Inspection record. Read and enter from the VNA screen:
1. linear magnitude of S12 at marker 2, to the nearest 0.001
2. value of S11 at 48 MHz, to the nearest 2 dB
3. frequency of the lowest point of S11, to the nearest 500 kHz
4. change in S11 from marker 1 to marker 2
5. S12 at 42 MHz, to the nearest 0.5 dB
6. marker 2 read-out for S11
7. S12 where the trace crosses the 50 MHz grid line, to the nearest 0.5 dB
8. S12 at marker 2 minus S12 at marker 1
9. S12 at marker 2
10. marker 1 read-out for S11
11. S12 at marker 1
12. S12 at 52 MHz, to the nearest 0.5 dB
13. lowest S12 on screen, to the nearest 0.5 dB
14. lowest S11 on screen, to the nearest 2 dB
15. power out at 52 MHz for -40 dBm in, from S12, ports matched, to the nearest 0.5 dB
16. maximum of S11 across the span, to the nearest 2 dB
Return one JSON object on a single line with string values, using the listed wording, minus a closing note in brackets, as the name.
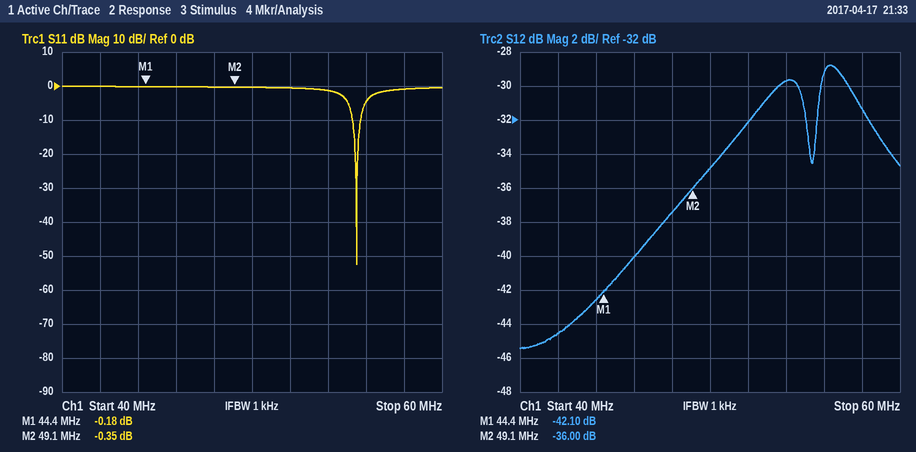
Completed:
{"linear magnitude of S12 at marker 2, to the nearest 0.001": "0.016", "value of S11 at 48 MHz, to the nearest 2 dB": "0 dB", "frequency of the lowest point of S11, to the nearest 500 kHz": "55.5 MHz", "change in S11 from marker 1 to marker 2": "-0.17 dB", "S12 at 42 MHz, to the nearest 0.5 dB": "-44.5 dB", "marker 2 read-out for S11": "-0.35 dB", "S12 where the trace crosses the 50 MHz grid line, to the nearest 0.5 dB": "-35.0 dB", "S12 at marker 2 minus S12 at marker 1": "6.10 dB", "S12 at marker 2": "-36.00 dB", "marker 1 read-out for S11": "-0.18 dB", "S12 at marker 1": "-42.10 dB", "S12 at 52 MHz, to the nearest 0.5 dB": "-32.0 dB", "lowest S12 on screen, to the nearest 0.5 dB": "-45.5 dB", "lowest S11 on screen, to the nearest 2 dB": "-52 dB", "power out at 52 MHz for -40 dBm in, from S12, ports matched, to the nearest 0.5 dB": "-72.0 dBm", "maximum of S11 across the span, to the nearest 2 dB": "0 dB"}
